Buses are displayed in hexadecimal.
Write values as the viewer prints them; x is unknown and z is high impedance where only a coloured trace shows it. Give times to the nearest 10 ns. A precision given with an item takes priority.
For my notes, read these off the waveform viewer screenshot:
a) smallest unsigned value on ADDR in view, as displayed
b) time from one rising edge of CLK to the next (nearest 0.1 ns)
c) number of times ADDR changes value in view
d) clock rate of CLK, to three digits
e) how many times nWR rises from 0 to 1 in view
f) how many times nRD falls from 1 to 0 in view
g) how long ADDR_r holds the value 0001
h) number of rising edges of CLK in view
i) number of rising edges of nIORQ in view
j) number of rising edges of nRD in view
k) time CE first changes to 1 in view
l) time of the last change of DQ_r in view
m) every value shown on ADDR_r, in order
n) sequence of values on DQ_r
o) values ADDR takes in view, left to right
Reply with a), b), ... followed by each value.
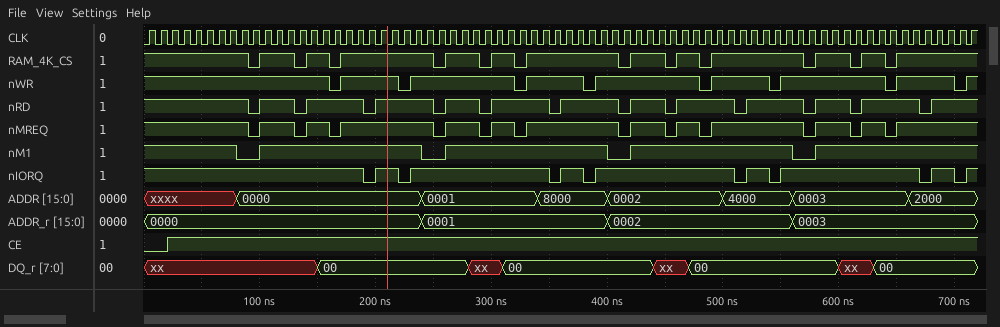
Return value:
a) 0000
b) 10 ns
c) 7
d) 100 MHz
e) 8
f) 12
g) 160 ns
h) 72
i) 8
j) 12
k) 20 ns
l) 630 ns
m) 0000, 0001, 0002, 0003
n) xx, 00, xx, 00, xx, 00, xx, 00
o) xxxx, 0000, 0001, 8000, 0002, 4000, 0003, 2000
